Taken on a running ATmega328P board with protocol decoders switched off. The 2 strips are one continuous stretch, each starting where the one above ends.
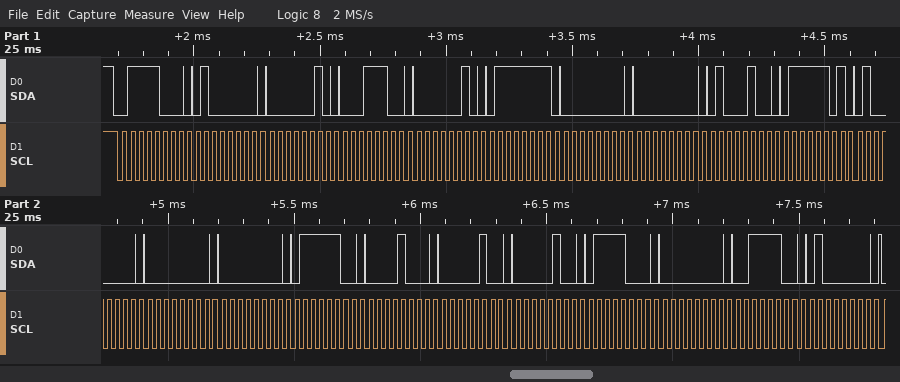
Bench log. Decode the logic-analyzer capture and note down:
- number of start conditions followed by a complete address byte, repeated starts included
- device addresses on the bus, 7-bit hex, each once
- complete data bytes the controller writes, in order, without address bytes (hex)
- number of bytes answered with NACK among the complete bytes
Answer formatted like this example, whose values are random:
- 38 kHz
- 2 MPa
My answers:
- 1
- 0x3C
- 40 02 1C 02 7F 00 00 44 7D 40 00 00 7C 08 04 04 78 00 3C 40
- 0
